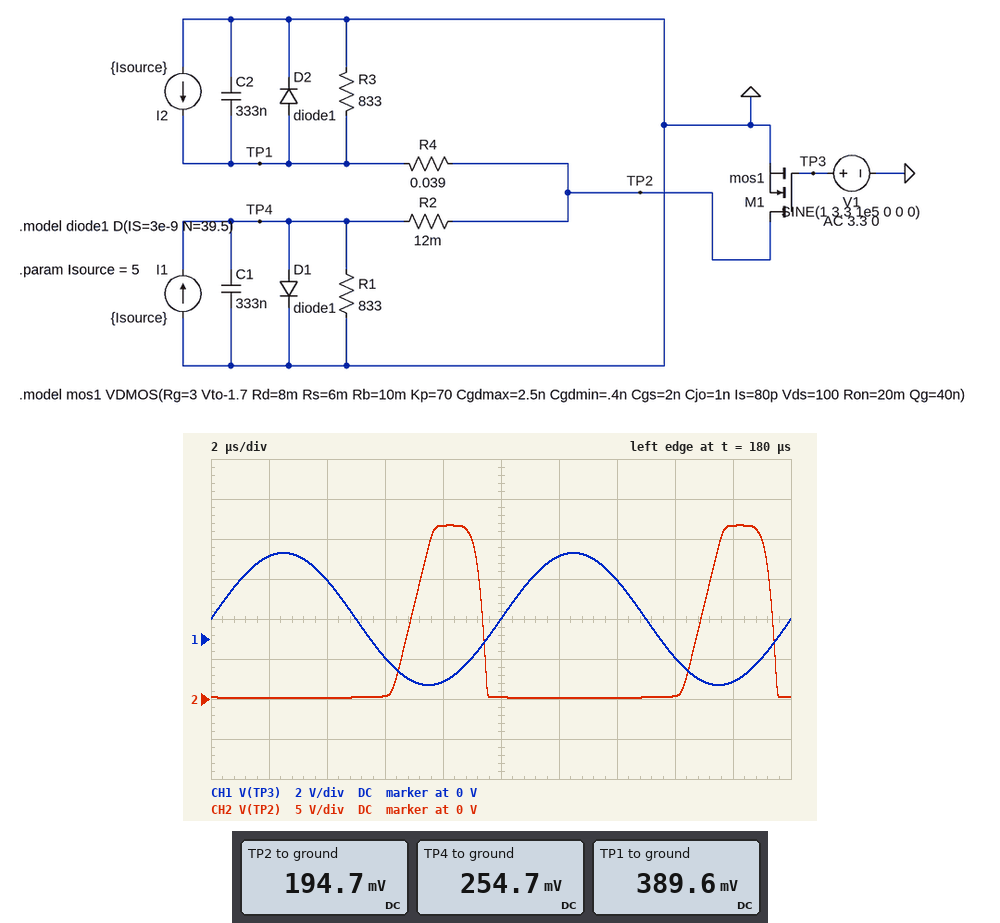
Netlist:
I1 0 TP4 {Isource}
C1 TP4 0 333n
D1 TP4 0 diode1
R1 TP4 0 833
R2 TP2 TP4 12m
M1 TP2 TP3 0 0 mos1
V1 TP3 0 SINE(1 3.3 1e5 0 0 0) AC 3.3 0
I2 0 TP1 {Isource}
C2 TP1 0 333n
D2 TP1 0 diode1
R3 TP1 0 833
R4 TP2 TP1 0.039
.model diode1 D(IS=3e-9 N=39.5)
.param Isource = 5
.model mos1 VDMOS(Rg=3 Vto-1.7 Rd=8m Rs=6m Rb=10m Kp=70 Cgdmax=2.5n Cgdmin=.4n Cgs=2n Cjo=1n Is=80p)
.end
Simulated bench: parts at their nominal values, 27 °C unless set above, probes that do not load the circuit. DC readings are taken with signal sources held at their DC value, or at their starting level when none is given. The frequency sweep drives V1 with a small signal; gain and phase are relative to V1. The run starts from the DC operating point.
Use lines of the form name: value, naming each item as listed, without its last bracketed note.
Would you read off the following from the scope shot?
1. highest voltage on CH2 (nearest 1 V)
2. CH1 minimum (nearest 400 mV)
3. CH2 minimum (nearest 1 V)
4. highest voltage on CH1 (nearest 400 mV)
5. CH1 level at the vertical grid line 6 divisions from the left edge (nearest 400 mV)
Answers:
highest voltage on CH2: 22 V
CH1 minimum: -2.4 V
CH2 minimum: 0 V
highest voltage on CH1: 4.4 V
CH1 level at the vertical grid line 6 divisions from the left edge: 4.0 V
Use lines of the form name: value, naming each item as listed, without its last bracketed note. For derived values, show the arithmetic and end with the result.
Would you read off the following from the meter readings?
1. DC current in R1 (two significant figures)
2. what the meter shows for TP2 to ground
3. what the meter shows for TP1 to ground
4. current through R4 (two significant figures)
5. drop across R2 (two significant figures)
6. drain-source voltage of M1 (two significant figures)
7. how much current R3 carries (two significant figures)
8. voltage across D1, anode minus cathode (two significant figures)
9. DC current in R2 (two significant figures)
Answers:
DC current in R1: (254.7 mV) / 833 Ω = 310 µA
what the meter shows for TP2 to ground: 194.7 mV
what the meter shows for TP1 to ground: 389.6 mV
current through R4: (389.6 mV - 194.7 mV) / 39 mΩ = 5.0 A
drop across R2: 254.7 mV - 194.7 mV = 60 mV
drain-source voltage of M1: 194.7 mV = 190 mV
how much current R3 carries: (389.6 mV) / 833 Ω = 470 µA
voltage across D1, anode minus cathode: 254.7 mV = 250 mV
DC current in R2: (254.7 mV - 194.7 mV) / 12 mΩ = 5.0 A
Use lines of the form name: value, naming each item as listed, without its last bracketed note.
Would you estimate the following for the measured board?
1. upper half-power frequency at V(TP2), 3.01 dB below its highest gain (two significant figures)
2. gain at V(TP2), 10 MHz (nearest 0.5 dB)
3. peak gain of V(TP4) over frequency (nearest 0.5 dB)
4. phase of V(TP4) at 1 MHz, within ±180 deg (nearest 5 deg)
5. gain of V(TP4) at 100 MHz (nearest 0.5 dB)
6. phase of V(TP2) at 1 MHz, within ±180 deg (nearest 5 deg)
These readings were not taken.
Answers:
upper half-power frequency at V(TP2), 3.01 dB below its highest gain: 6.6 MHz
gain at V(TP2), 10 MHz: -39.0 dB
peak gain of V(TP4) over frequency: -33.5 dB
phase of V(TP4) at 1 MHz, within ±180 deg: 170 deg
gain of V(TP4) at 100 MHz: -66.0 dB
phase of V(TP2) at 1 MHz, within ±180 deg: 170 deg
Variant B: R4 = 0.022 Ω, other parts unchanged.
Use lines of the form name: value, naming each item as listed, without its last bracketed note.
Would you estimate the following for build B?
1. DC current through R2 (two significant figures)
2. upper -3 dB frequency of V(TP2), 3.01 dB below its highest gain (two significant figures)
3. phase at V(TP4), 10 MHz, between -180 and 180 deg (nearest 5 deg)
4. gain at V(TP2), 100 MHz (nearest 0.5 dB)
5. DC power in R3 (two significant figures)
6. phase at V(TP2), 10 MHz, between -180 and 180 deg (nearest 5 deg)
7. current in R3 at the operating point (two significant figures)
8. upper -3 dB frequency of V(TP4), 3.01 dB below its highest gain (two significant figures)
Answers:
DC current through R2: 5.0 A
upper -3 dB frequency of V(TP2), 3.01 dB below its highest gain: 6.8 MHz
phase at V(TP4), 10 MHz, between -180 and 180 deg: 90 deg
gain at V(TP2), 100 MHz: -58.5 dB
DC power in R3: 110 µW
phase at V(TP2), 10 MHz, between -180 and 180 deg: 105 deg
current in R3 at the operating point: 370 µA
upper -3 dB frequency of V(TP4), 3.01 dB below its highest gain: 6.6 MHz
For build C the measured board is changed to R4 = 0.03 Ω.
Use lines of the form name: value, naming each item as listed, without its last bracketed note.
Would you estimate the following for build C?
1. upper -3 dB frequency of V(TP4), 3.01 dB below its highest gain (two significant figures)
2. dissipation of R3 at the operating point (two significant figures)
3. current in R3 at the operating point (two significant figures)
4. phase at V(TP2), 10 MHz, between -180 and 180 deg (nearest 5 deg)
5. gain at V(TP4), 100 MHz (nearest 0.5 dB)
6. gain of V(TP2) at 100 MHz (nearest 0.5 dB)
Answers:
upper -3 dB frequency of V(TP4), 3.01 dB below its highest gain: 6.5 MHz
dissipation of R3 at the operating point: 140 µW
current in R3 at the operating point: 410 µA
phase at V(TP2), 10 MHz, between -180 and 180 deg: 105 deg
gain at V(TP4), 100 MHz: -66.5 dB
gain of V(TP2) at 100 MHz: -58.0 dB
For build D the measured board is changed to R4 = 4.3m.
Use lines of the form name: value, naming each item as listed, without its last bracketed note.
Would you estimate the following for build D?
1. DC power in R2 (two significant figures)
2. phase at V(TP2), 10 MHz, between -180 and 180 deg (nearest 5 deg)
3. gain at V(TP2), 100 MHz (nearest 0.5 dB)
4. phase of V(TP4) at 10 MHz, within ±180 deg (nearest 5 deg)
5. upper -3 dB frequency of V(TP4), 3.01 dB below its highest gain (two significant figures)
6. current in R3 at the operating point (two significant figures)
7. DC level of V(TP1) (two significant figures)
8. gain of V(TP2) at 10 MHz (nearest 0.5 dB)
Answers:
DC power in R2: 300 mW
phase at V(TP2), 10 MHz, between -180 and 180 deg: 100 deg
gain at V(TP2), 100 MHz: -62.5 dB
phase of V(TP4) at 10 MHz, within ±180 deg: 85 deg
upper -3 dB frequency of V(TP4), 3.01 dB below its highest gain: 7.0 MHz
current in R3 at the operating point: 260 µA
DC level of V(TP1): 220 mV
gain of V(TP2) at 10 MHz: -38.5 dB
